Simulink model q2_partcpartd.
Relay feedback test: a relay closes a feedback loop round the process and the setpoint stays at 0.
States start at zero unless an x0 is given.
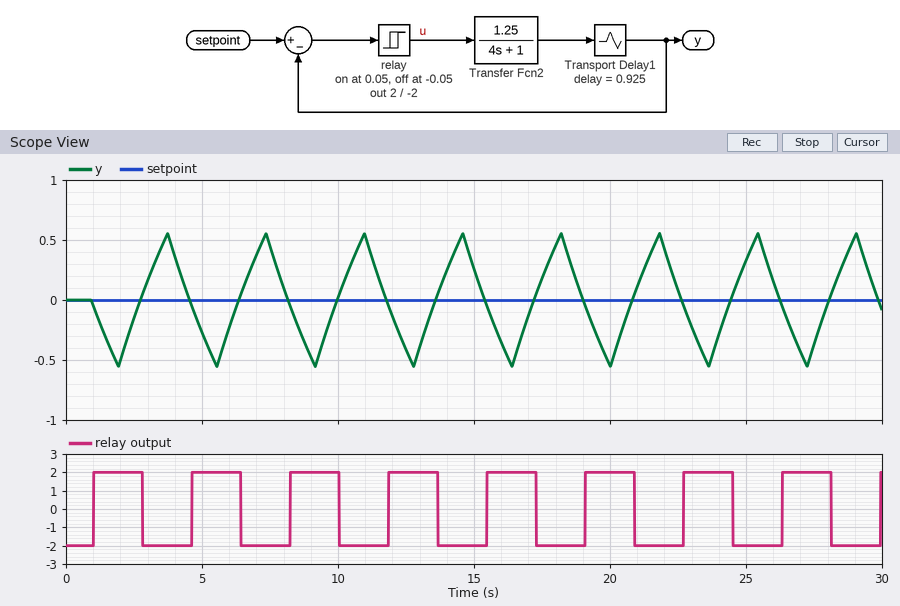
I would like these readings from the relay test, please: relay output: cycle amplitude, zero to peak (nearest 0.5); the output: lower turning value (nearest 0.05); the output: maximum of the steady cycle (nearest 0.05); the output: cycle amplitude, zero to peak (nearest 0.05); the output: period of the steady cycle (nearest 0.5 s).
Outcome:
2.0
-0.55
0.55
0.55
3.5 s
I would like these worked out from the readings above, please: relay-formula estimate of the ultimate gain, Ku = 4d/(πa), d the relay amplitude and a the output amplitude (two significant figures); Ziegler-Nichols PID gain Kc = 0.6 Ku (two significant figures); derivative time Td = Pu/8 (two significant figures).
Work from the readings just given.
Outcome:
4.6
2.8
0.44 s
